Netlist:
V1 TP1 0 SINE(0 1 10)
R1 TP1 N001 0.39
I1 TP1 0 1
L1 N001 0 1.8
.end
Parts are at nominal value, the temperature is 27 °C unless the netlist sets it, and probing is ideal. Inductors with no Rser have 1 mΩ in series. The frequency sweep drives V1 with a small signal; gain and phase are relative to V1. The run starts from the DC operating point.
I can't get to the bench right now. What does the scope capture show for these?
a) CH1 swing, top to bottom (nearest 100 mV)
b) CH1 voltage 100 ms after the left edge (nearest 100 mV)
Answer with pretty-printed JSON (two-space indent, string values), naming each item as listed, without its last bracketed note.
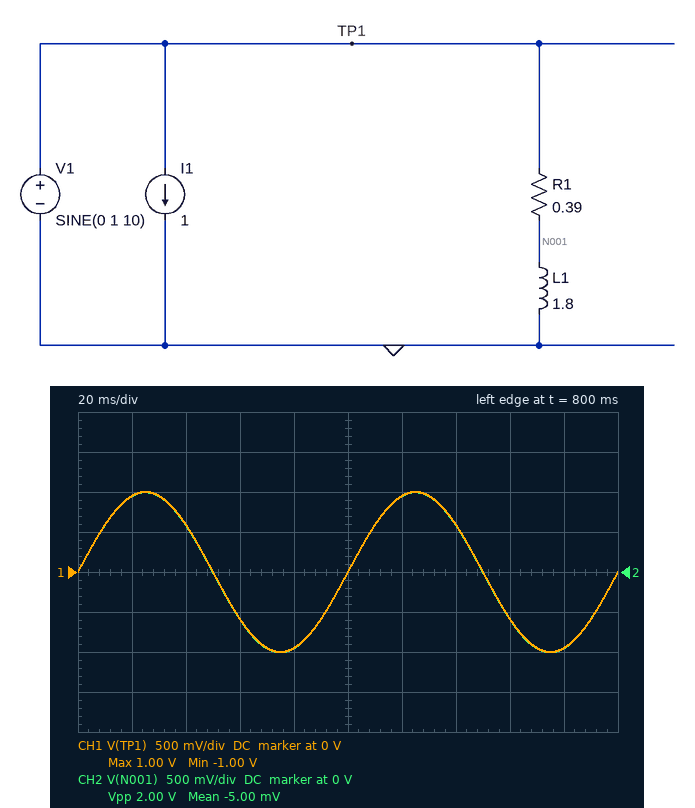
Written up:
{
  "CH1 swing, top to bottom": "2.0 V",
  "CH1 voltage 100 ms after the left edge": "0 V"
}
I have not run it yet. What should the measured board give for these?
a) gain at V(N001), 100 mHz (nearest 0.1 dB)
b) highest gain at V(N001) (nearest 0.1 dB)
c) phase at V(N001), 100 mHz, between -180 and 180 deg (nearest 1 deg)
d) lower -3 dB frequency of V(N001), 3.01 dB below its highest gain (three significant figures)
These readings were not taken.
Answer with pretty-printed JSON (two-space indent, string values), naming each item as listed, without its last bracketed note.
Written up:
{
  "gain at V(N001), 100 mHz": "-0.5 dB",
  "highest gain at V(N001)": "0 dB",
  "phase at V(N001), 100 mHz, between -180 and 180 deg": "19 deg",
  "lower -3 dB frequency of V(N001), 3.01 dB below its highest gain": "34.6 mHz"
}
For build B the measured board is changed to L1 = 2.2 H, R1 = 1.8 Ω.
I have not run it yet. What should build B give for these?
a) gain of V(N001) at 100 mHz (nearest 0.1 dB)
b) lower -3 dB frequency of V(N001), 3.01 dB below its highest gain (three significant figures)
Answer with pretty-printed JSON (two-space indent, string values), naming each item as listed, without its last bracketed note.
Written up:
{
  "gain of V(N001) at 100 mHz": "-4.3 dB",
  "lower -3 dB frequency of V(N001), 3.01 dB below its highest gain": "130 mHz"
}
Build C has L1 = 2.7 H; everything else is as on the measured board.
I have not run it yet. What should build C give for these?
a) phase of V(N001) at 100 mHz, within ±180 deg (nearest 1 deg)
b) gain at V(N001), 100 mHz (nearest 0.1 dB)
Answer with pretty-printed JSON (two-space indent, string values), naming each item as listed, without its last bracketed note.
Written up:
{
  "phase of V(N001) at 100 mHz, within ±180 deg": "13 deg",
  "gain at V(N001), 100 mHz": "-0.2 dB"
}
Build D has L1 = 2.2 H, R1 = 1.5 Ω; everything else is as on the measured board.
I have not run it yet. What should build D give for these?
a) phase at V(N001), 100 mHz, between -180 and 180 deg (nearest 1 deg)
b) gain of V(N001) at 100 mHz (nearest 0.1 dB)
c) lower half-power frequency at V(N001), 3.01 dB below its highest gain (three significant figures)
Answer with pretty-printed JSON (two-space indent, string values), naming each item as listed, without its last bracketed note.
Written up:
{
  "phase at V(N001), 100 mHz, between -180 and 180 deg": "47 deg",
  "gain of V(N001) at 100 mHz": "-3.4 dB",
  "lower half-power frequency at V(N001), 3.01 dB below its highest gain": "109 mHz"
}
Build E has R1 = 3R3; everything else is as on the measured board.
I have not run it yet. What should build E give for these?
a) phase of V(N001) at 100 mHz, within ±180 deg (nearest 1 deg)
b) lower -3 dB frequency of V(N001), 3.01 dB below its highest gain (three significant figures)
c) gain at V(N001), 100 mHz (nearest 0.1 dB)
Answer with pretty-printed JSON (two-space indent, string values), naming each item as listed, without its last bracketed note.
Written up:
{
  "phase of V(N001) at 100 mHz, within ±180 deg": "71 deg",
  "lower -3 dB frequency of V(N001), 3.01 dB below its highest gain": "292 mHz",
  "gain at V(N001), 100 mHz": "-9.8 dB"
}
